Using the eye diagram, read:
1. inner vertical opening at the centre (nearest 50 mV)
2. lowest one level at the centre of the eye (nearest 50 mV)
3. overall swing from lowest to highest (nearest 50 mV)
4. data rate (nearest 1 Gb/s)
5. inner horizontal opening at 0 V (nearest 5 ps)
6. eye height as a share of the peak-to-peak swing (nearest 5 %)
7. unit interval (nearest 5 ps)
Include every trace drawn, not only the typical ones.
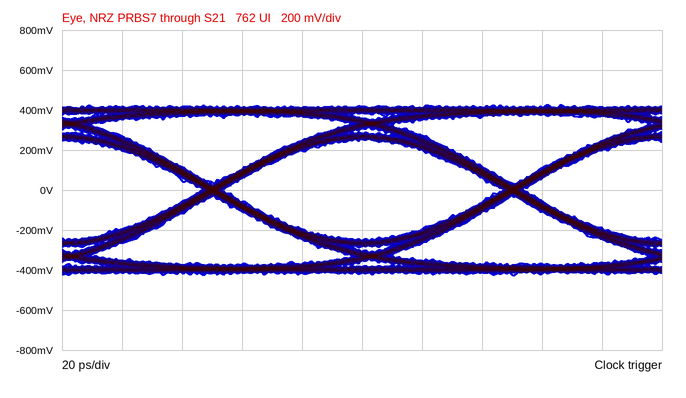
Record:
500 mV
250 mV
850 mV
10 Gb/s
95 ps
60 %
100 ps
